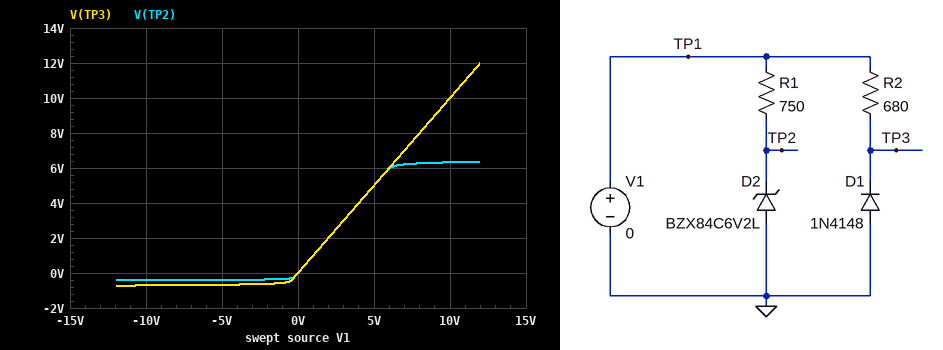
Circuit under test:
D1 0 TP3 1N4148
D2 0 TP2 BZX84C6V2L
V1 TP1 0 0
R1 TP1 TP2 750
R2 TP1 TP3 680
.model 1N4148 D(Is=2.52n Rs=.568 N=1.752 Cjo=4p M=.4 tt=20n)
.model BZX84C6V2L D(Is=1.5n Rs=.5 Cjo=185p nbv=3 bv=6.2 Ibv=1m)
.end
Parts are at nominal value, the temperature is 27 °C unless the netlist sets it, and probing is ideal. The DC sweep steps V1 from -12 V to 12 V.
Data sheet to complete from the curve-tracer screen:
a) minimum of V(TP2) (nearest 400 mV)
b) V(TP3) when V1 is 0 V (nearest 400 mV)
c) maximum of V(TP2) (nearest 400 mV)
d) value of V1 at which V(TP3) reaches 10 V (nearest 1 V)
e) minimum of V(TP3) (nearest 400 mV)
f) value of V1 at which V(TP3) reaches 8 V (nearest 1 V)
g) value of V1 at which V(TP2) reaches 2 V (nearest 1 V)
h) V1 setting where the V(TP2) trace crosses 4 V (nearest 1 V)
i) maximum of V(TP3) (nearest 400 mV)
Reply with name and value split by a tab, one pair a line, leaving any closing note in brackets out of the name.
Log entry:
minimum of V(TP2)	-400 mV
V(TP3) when V1 is 0 V	0 V
maximum of V(TP2)	6.4 V
value of V1 at which V(TP3) reaches 10 V	10 V
minimum of V(TP3)	-800 mV
value of V1 at which V(TP3) reaches 8 V	8 V
value of V1 at which V(TP2) reaches 2 V	2 V
V1 setting where the V(TP2) trace crosses 4 V	4 V
maximum of V(TP3)	12.0 V
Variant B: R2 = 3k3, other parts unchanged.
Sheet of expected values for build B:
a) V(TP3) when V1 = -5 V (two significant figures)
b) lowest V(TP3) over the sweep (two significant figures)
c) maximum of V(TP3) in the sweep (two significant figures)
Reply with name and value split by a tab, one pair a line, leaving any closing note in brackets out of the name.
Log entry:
V(TP3) when V1 = -5 V	-600 mV
lowest V(TP3) over the sweep	-640 mV
maximum of V(TP3) in the sweep	12 V
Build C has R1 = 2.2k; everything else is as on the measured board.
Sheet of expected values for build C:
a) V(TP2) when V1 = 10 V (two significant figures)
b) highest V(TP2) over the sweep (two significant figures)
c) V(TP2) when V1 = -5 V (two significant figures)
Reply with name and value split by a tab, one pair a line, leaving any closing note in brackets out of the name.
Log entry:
V(TP2) when V1 = 10 V	6.2 V
highest V(TP2) over the sweep	6.3 V
V(TP2) when V1 = -5 V	-370 mV
